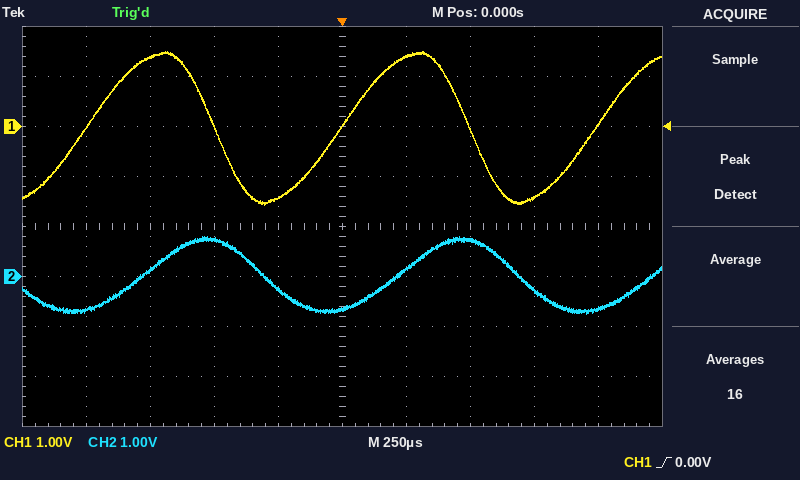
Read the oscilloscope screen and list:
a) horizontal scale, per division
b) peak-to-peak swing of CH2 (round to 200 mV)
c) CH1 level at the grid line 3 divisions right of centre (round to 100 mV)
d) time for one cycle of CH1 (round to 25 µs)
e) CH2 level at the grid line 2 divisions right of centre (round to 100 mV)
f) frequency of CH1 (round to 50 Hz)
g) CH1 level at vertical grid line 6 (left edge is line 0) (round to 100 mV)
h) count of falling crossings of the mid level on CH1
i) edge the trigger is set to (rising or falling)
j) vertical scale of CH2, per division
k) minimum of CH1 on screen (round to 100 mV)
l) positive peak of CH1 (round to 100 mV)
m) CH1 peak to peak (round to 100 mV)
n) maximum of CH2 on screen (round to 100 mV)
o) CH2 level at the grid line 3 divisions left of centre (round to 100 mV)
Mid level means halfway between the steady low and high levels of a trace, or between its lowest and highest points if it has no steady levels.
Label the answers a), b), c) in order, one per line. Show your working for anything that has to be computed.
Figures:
a) 250 µs
b) 1.6 V
c) -1.4 V
d) 1.000 ms
e) 700 mV
f) 1 / 1.000 ms ≈ 1.00 kHz
g) 1.4 V
h) 2
i) rising
j) 1 V
k) -1.6 V
l) 1.5 V
m) 1.5 V − (-1.6 V) = 3.1 V
n) 800 mV
o) 100 mV
